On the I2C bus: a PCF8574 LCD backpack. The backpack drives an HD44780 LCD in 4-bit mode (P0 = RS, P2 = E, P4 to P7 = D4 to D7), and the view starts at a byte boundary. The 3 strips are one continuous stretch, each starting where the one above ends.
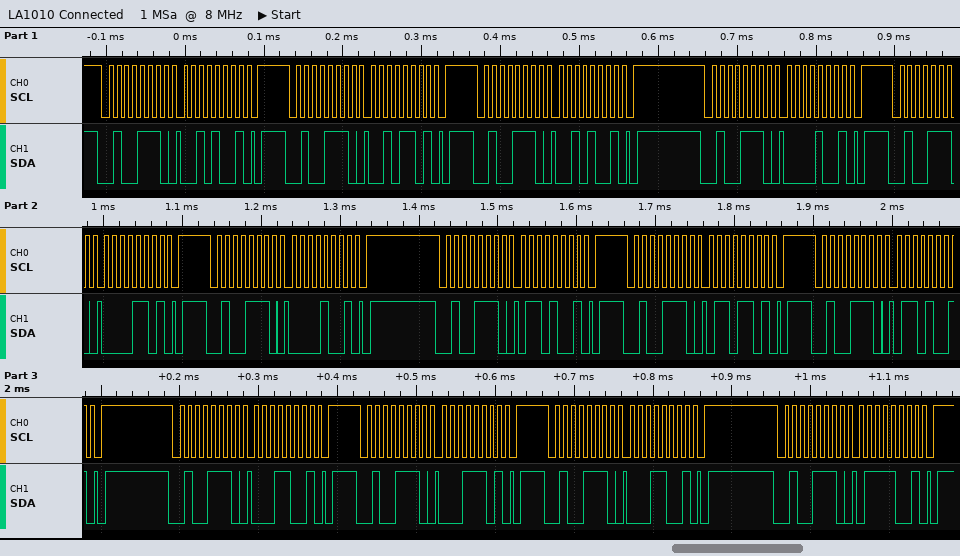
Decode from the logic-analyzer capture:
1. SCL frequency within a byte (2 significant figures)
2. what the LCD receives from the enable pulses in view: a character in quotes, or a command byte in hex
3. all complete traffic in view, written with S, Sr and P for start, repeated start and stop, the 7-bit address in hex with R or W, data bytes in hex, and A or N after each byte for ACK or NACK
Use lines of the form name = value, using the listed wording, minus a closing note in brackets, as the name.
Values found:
SCL frequency within a byte = 100 kHz
what the LCD receives from the enable pulses in view: a character in quotes, or a command byte in hex = ' ' 'a'
all complete traffic in view, written with S, Sr and P for start, repeated start and stop, the 7-bit address in hex with R or W, data bytes in hex, and A or N after each byte for ACK or NACK = S 27W A 29 A P S 27W A 2D A P S 27W A 29 A P S 27W A 09 A P S 27W A 0D A P S 27W A 09 A P S 27W A 69 A P S 27W A 6D A P S 27W A 69 A P S 27W A 19 A P S 27W A 1D A P S 27W A 19 A P S 27W A 79 A P
